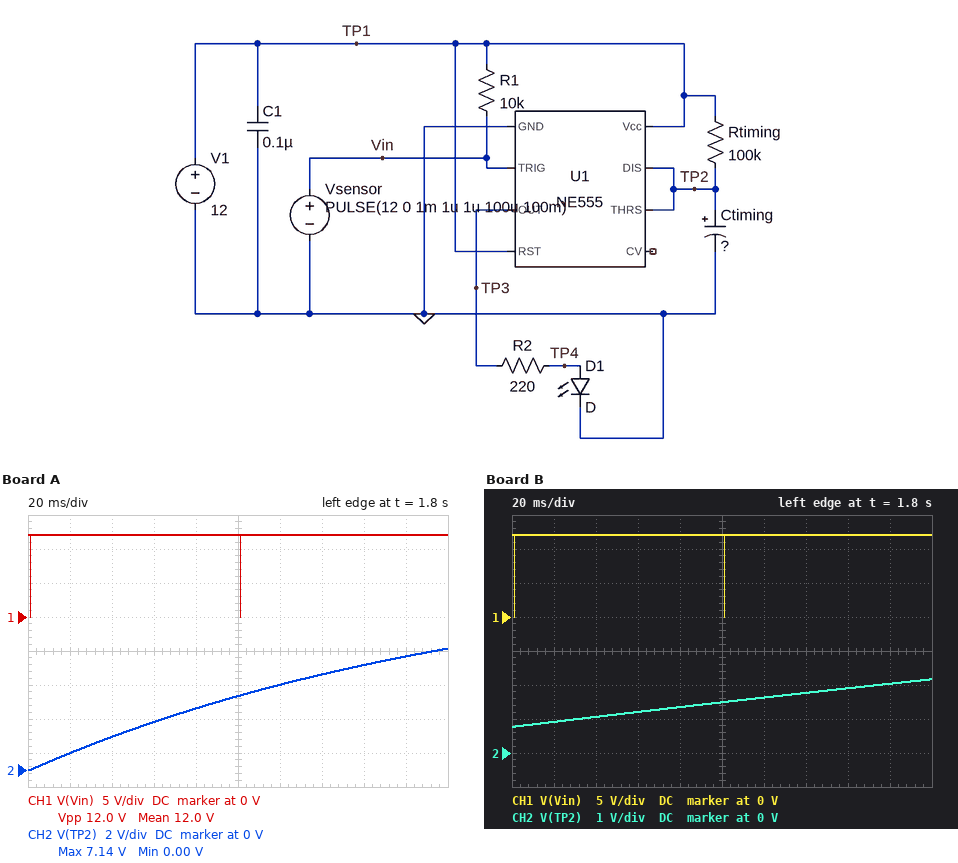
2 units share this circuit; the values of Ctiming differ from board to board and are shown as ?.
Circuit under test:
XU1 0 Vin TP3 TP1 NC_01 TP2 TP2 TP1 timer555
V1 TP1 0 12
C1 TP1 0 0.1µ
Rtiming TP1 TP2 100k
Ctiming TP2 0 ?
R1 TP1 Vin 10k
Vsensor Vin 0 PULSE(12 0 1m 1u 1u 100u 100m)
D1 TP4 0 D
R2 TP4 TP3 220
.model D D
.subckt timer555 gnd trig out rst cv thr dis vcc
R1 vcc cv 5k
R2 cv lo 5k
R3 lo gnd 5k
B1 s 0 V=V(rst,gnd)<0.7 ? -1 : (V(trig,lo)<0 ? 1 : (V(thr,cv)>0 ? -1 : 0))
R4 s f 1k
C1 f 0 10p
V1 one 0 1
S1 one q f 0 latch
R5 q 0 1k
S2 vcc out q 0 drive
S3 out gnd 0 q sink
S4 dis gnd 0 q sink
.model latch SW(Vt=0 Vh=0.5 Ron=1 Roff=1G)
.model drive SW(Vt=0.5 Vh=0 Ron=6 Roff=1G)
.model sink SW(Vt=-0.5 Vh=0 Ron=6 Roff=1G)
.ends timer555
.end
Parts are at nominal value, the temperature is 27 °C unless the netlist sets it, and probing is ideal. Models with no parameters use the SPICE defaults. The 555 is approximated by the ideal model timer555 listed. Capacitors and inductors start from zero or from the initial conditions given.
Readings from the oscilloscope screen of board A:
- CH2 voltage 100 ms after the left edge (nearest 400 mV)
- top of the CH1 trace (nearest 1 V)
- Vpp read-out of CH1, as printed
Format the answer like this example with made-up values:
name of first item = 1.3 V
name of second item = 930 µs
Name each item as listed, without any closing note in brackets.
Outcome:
CH2 voltage 100 ms after the left edge = 4.4 V
top of the CH1 trace = 12 V
Vpp read-out of CH1, as printed = 12.0 V
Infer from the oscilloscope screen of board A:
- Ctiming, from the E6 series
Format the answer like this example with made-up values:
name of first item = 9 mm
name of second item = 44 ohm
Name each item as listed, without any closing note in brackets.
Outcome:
Ctiming, from the E6 series = 2.2 µF
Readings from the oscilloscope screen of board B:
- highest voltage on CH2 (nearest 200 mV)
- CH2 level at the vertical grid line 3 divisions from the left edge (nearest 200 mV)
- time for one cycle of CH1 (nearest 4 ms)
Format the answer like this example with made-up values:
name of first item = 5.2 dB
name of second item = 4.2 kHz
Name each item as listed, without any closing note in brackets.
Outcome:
highest voltage on CH2 = 2.2 V
CH2 level at the vertical grid line 3 divisions from the left edge = 1.2 V
time for one cycle of CH1 = 100 ms
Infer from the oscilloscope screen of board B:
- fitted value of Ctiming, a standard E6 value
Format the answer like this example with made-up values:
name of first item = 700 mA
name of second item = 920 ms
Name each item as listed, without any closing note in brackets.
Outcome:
fitted value of Ctiming, a standard E6 value = 15 µF
